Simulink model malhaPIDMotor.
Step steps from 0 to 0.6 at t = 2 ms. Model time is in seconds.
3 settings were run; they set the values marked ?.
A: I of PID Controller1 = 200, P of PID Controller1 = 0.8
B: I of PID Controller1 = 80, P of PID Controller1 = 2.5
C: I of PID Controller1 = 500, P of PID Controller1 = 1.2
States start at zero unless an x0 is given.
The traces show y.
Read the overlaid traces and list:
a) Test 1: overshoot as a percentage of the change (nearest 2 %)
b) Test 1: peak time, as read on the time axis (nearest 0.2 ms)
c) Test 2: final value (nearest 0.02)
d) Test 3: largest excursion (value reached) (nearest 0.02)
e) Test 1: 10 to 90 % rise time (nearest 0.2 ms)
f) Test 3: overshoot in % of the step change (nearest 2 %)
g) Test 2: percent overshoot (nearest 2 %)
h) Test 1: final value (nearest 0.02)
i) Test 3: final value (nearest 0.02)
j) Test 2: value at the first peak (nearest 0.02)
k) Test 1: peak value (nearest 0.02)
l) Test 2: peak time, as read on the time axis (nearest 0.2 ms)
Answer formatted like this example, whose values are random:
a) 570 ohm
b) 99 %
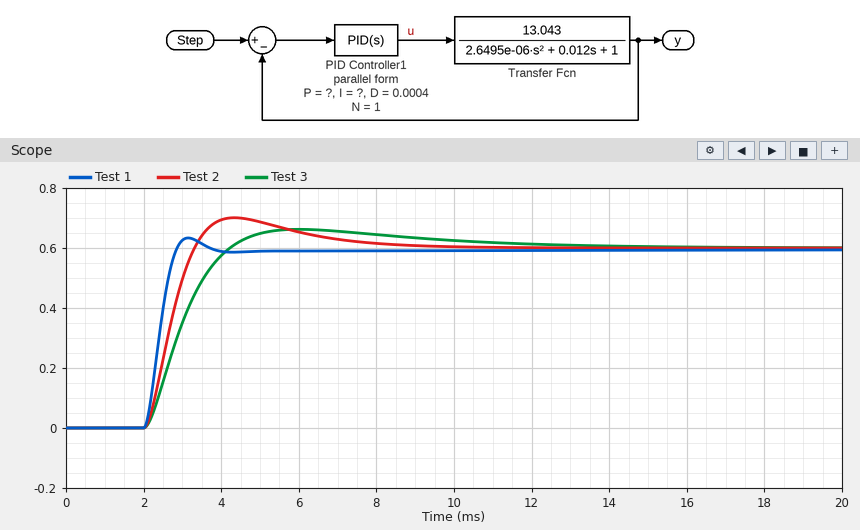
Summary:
a) 6 %
b) 3.2 ms
c) 0.60
d) 0.66
e) 0.6 ms
f) 10 %
g) 16 %
h) 0.60
i) 0.60
j) 0.70
k) 0.64
l) 4.4 ms
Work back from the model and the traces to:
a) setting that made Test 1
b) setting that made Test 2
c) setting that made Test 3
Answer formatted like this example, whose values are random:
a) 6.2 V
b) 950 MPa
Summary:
a) B
b) C
c) A
